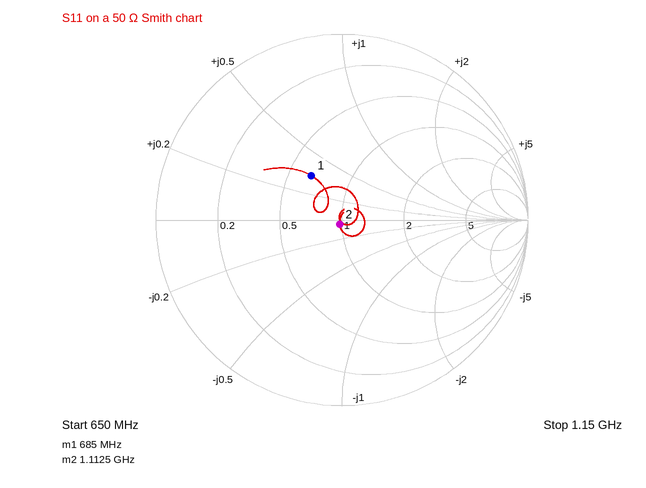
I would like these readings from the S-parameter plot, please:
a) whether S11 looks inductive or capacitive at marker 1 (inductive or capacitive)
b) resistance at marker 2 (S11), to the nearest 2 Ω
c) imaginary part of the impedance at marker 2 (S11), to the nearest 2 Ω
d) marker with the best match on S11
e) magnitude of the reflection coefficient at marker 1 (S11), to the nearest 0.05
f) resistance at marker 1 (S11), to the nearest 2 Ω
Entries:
inductive
48 Ω
-2 Ω
marker 2
0.30
32 Ω
